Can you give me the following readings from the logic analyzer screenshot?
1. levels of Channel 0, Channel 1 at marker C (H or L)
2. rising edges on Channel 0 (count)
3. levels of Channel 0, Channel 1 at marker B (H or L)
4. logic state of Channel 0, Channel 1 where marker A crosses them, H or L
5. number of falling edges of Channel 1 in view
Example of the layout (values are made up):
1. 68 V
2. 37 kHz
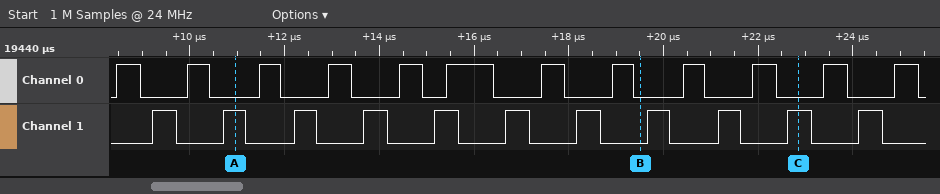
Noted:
1. Channel 0=L, Channel 1=H
2. 12
3. Channel 0=L, Channel 1=L
4. Channel 0=L, Channel 1=H
5. 11
